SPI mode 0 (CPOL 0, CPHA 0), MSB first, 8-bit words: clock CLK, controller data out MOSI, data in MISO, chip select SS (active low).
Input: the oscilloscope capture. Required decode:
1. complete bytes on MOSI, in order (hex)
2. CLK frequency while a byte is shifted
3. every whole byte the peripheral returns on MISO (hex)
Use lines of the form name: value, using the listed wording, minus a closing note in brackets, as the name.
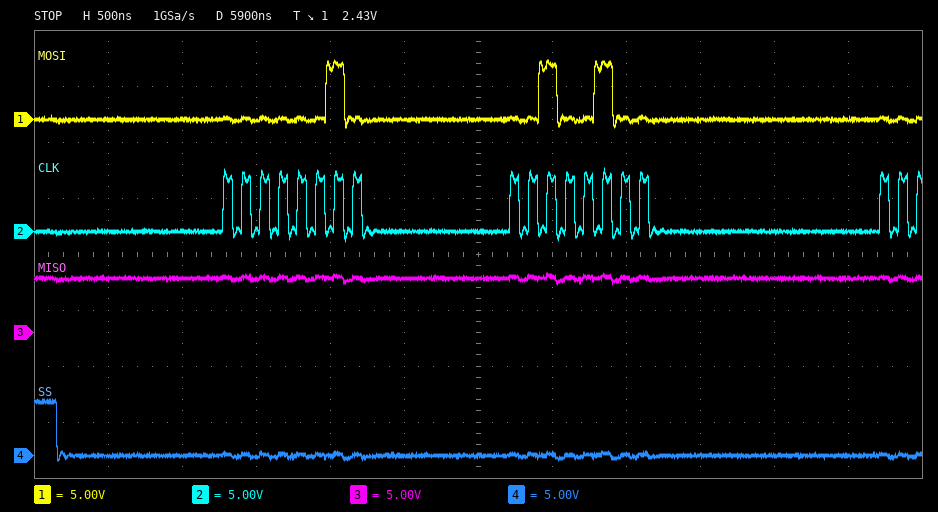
complete bytes on MOSI, in order: 02 24
CLK frequency while a byte is shifted: 8 MHz
every whole byte the peripheral returns on MISO: FF FF
